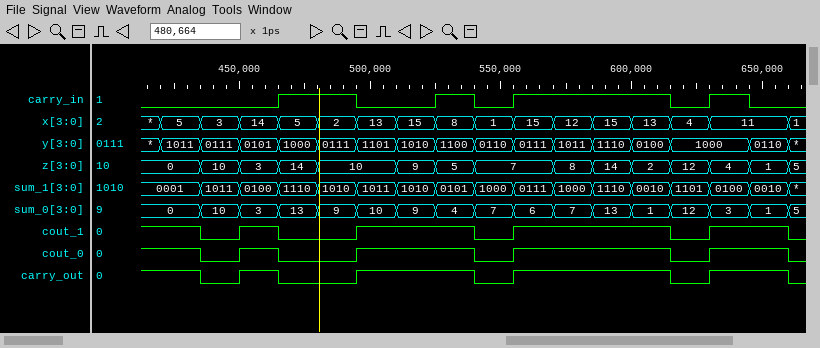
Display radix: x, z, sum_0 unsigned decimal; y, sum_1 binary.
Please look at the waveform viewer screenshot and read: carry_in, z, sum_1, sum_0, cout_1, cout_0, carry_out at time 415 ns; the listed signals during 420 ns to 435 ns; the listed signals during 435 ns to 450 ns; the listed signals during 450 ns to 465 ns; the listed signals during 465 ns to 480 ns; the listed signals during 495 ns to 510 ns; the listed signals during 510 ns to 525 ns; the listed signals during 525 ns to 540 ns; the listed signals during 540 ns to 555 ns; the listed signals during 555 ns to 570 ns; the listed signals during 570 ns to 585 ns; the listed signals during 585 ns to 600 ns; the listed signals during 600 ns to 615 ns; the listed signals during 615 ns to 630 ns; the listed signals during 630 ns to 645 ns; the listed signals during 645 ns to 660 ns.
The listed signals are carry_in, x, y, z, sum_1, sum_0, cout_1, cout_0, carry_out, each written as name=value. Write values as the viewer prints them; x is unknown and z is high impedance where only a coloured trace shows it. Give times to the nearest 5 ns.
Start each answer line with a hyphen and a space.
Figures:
- carry_in=0, z=0, sum_1=0001, sum_0=0, cout_1=1, cout_0=1, carry_out=1
- carry_in=0, x=5, y=1011, z=0, sum_1=0001, sum_0=0, cout_1=1, cout_0=1, carry_out=1
- carry_in=0, x=3, y=0111, z=10, sum_1=1011, sum_0=10, cout_1=0, cout_0=0, carry_out=0
- carry_in=0, x=14, y=0101, z=3, sum_1=0100, sum_0=3, cout_1=1, cout_0=1, carry_out=1
- carry_in=1, x=5, y=1000, z=14, sum_1=1110, sum_0=13, cout_1=0, cout_0=0, carry_out=0
- carry_in=0, x=13, y=1101, z=10, sum_1=1011, sum_0=10, cout_1=1, cout_0=1, carry_out=1
- carry_in=0, x=15, y=1010, z=9, sum_1=1010, sum_0=9, cout_1=1, cout_0=1, carry_out=1
- carry_in=1, x=8, y=1100, z=5, sum_1=0101, sum_0=4, cout_1=1, cout_0=1, carry_out=1
- carry_in=0, x=1, y=0110, z=7, sum_1=1000, sum_0=7, cout_1=0, cout_0=0, carry_out=0
- carry_in=1, x=15, y=0111, z=7, sum_1=0111, sum_0=6, cout_1=1, cout_0=1, carry_out=1
- carry_in=1, x=12, y=1011, z=8, sum_1=1000, sum_0=7, cout_1=1, cout_0=1, carry_out=1
- carry_in=1, x=15, y=1110, z=14, sum_1=1110, sum_0=13, cout_1=1, cout_0=1, carry_out=1
- carry_in=1, x=13, y=0100, z=2, sum_1=0010, sum_0=1, cout_1=1, cout_0=1, carry_out=1
- carry_in=0, x=4, y=1000, z=12, sum_1=1101, sum_0=12, cout_1=0, cout_0=0, carry_out=0
- carry_in=1, x=11, y=1000, z=4, sum_1=0100, sum_0=3, cout_1=1, cout_0=1, carry_out=1
- carry_in=0, x=11, y=0110, z=1, sum_1=0010, sum_0=1, cout_1=1, cout_0=1, carry_out=1
